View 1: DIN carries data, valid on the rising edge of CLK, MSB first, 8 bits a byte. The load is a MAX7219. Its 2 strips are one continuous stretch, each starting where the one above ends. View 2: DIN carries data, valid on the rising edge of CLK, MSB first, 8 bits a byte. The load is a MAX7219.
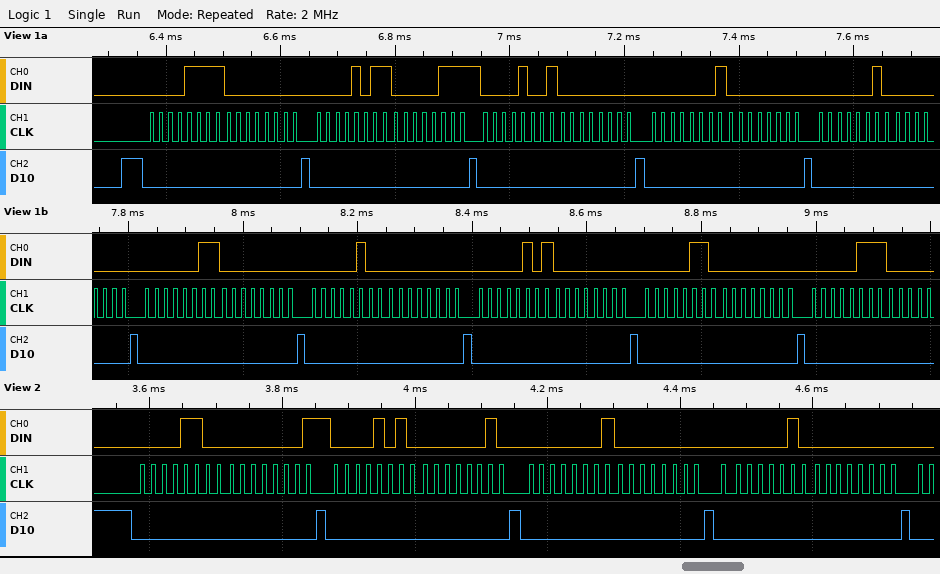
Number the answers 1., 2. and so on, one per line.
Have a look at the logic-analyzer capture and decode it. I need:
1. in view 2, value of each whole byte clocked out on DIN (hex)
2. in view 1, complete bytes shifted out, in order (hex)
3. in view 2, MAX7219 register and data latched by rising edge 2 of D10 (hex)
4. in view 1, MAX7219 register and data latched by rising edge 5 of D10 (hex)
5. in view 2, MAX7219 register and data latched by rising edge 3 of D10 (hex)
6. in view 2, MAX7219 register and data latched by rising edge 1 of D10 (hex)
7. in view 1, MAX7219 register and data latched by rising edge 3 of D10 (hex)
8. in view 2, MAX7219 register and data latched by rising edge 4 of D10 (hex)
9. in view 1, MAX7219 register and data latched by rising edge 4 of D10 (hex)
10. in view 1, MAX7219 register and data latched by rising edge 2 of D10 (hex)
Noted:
1. 0C 01 0A 02 01 00 02 00
2. 0F 00 0B 07 09 00 01 00 02 00 03 00 04 00 05 00 06 00 07
3. register 0xA, data 0x02
4. register 0x1, data 0x00
5. register 0x1, data 0x00
6. register 0xC, data 0x01
7. register 0xB, data 0x07
8. register 0x2, data 0x00
9. register 0x9, data 0x00
10. register 0xF, data 0x00
